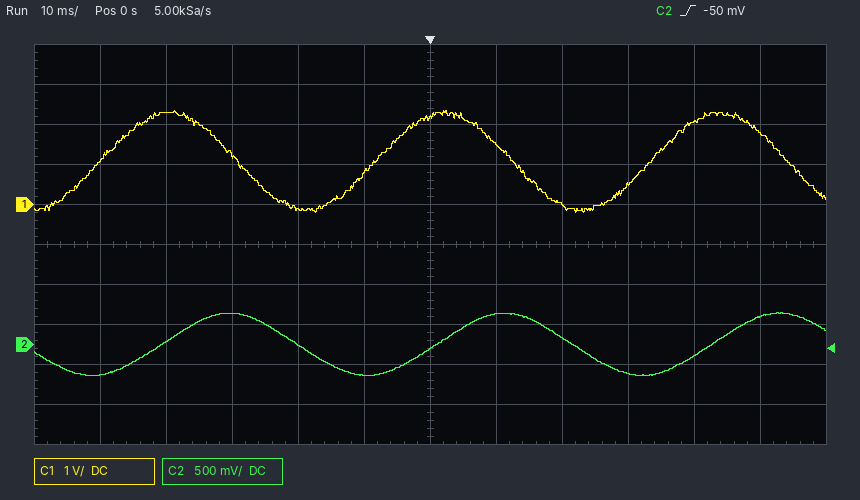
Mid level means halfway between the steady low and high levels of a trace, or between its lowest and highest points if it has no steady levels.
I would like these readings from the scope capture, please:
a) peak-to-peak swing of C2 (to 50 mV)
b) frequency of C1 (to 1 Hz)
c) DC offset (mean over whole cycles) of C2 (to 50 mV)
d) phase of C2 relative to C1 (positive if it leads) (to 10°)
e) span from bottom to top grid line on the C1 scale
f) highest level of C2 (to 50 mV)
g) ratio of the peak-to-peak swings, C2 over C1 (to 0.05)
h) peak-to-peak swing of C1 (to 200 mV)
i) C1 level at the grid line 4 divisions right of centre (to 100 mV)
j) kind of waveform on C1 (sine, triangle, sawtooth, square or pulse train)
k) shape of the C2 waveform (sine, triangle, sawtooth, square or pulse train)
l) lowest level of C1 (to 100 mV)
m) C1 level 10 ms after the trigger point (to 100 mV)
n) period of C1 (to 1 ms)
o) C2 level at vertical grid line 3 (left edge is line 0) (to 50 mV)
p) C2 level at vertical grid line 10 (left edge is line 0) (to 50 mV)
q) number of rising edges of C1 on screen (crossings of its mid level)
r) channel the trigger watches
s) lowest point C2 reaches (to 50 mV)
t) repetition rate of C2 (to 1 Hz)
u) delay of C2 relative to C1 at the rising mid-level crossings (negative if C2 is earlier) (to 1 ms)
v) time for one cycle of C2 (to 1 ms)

800 mV
24 Hz
0 mV
-80°
10 V
400 mV
0.30
2.6 V
2.1 V
sine
sine
-200 mV
1.5 V
42 ms
400 mV
-150 mV
3
C2
-400 mV
24 Hz
+9 ms
42 ms
